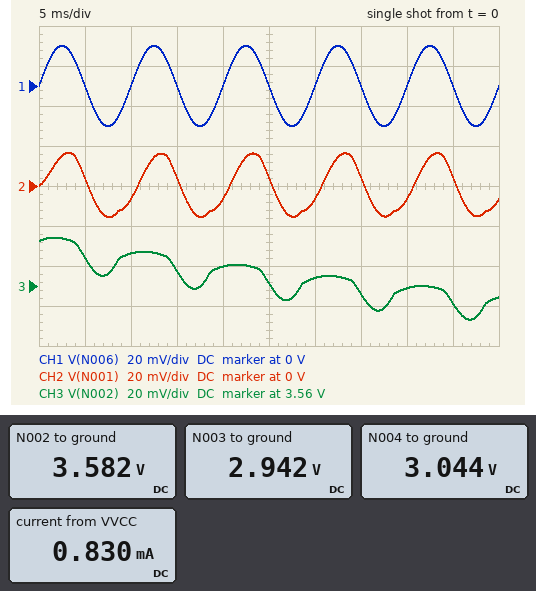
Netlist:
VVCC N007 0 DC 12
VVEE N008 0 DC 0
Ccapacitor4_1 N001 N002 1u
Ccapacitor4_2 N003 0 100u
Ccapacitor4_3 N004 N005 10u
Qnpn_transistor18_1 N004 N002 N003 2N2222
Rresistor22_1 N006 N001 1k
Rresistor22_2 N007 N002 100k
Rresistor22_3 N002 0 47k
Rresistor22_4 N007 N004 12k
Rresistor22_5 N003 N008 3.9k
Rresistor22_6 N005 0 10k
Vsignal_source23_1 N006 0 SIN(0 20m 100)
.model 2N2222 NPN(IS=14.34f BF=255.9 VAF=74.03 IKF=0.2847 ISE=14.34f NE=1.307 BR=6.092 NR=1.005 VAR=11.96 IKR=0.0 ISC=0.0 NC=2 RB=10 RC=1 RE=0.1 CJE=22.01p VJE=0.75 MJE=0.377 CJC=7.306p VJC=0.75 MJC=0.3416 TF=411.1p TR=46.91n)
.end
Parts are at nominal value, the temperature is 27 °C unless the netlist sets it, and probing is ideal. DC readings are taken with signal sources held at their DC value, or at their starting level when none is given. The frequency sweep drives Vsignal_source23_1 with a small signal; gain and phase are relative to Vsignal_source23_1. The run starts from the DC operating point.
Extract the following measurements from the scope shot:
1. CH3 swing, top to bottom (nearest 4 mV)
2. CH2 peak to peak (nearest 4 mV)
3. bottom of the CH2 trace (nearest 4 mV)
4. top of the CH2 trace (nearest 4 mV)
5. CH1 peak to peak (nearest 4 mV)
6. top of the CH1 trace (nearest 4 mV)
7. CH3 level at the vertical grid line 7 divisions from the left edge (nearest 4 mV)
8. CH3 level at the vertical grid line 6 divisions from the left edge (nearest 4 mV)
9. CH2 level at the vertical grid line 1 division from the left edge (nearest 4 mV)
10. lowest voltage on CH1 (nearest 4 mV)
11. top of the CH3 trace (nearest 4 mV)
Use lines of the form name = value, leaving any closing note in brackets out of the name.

CH3 swing, top to bottom = 40 mV
CH2 peak to peak = 32 mV
bottom of the CH2 trace = -16 mV
top of the CH2 trace = 16 mV
CH1 peak to peak = 40 mV
top of the CH1 trace = 20 mV
CH3 level at the vertical grid line 7 divisions from the left edge = 3.556 V
CH3 level at the vertical grid line 6 divisions from the left edge = 3.564 V
CH2 level at the vertical grid line 1 division from the left edge = 4 mV
lowest voltage on CH1 = -20 mV
top of the CH3 trace = 3.584 V
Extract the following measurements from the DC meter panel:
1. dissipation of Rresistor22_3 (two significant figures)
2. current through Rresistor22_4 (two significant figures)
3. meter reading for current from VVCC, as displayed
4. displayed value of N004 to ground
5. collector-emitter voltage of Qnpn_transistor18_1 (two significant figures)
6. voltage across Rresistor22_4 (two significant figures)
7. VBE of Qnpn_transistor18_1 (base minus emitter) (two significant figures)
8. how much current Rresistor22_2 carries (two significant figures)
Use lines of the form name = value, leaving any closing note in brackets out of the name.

dissipation of Rresistor22_3 = 270 µW
current through Rresistor22_4 = 750 µA
meter reading for current from VVCC, as displayed = 0.830 mA
displayed value of N004 to ground = 3.044 V
collector-emitter voltage of Qnpn_transistor18_1 = 100 mV
voltage across Rresistor22_4 = 9.0 V
VBE of Qnpn_transistor18_1 (base minus emitter) = 640 mV
how much current Rresistor22_2 carries = 84 µA
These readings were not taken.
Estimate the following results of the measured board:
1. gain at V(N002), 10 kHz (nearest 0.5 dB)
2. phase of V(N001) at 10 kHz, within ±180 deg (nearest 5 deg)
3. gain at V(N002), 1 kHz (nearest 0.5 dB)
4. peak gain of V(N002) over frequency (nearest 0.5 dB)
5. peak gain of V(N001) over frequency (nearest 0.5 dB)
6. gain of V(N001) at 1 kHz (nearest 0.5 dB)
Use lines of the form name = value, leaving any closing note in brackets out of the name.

gain at V(N002), 10 kHz = -13.0 dB
phase of V(N001) at 10 kHz, within ±180 deg = -5 deg
gain at V(N002), 1 kHz = -13.0 dB
peak gain of V(N002) over frequency = -13.0 dB
peak gain of V(N001) over frequency = 0 dB
gain of V(N001) at 1 kHz = -12.0 dB
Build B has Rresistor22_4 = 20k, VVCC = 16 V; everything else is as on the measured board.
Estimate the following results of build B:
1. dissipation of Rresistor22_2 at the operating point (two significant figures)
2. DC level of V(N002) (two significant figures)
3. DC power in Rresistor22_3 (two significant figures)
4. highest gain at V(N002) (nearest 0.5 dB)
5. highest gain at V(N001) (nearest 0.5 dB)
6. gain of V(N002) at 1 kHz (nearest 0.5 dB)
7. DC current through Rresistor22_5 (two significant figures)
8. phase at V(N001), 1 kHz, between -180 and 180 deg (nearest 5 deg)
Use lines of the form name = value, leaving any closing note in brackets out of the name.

dissipation of Rresistor22_2 at the operating point = 1.6 mW
DC level of V(N002) = 3.4 V
DC power in Rresistor22_3 = 250 µW
highest gain at V(N002) = -16.0 dB
highest gain at V(N001) = 0 dB
gain of V(N002) at 1 kHz = -16.5 dB
DC current through Rresistor22_5 = 710 µA
phase at V(N001), 1 kHz, between -180 and 180 deg = -35 deg
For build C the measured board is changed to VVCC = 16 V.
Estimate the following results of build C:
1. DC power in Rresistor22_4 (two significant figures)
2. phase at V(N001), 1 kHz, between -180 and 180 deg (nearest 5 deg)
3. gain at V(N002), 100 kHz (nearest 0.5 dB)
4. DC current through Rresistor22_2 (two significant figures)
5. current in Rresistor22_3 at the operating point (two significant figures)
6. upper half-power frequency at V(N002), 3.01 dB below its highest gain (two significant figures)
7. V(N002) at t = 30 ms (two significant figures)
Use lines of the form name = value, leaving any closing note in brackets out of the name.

DC power in Rresistor22_4 = 12 mW
phase at V(N001), 1 kHz, between -180 and 180 deg = -35 deg
gain at V(N002), 100 kHz = -16.5 dB
DC current through Rresistor22_2 = 110 µA
current in Rresistor22_3 at the operating point = 98 µA
upper half-power frequency at V(N002), 3.01 dB below its highest gain = 610 kHz
V(N002) at t = 30 ms = 4.6 V
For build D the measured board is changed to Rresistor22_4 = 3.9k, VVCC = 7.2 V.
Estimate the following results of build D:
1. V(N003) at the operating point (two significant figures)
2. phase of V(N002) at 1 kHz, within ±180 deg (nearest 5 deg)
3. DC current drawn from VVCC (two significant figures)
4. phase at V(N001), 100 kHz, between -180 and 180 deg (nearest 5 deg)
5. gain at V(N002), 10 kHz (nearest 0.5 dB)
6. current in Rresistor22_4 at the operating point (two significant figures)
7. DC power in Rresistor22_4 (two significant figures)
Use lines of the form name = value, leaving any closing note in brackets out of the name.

V(N003) at the operating point = 1.6 V
phase of V(N002) at 1 kHz, within ±180 deg = 0 deg
DC current drawn from VVCC = 450 µA
phase at V(N001), 100 kHz, between -180 and 180 deg = -5 deg
gain at V(N002), 10 kHz = -1.0 dB
current in Rresistor22_4 at the operating point = 400 µA
DC power in Rresistor22_4 = 630 µW
